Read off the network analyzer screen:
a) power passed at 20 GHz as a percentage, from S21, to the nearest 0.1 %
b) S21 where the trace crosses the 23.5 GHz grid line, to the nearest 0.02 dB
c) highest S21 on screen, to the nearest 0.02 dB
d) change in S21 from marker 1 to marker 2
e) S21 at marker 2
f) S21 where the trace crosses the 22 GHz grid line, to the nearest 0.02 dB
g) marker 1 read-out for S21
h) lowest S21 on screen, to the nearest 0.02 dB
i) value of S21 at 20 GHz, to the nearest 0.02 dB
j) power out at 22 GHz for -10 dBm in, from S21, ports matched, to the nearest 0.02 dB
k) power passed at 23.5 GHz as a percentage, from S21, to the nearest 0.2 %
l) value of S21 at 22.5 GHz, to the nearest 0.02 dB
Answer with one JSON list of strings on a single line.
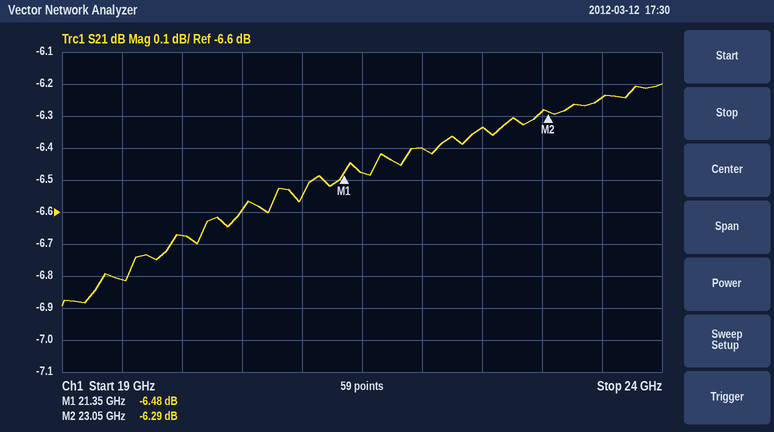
["21.5 %", "-6.24 dB", "-6.20 dB", "0.19 dB", "-6.29 dB", "-6.40 dB", "-6.48 dB", "-6.90 dB", "-6.68 dB", "-16.40 dBm", "23.8 %", "-6.34 dB"]
